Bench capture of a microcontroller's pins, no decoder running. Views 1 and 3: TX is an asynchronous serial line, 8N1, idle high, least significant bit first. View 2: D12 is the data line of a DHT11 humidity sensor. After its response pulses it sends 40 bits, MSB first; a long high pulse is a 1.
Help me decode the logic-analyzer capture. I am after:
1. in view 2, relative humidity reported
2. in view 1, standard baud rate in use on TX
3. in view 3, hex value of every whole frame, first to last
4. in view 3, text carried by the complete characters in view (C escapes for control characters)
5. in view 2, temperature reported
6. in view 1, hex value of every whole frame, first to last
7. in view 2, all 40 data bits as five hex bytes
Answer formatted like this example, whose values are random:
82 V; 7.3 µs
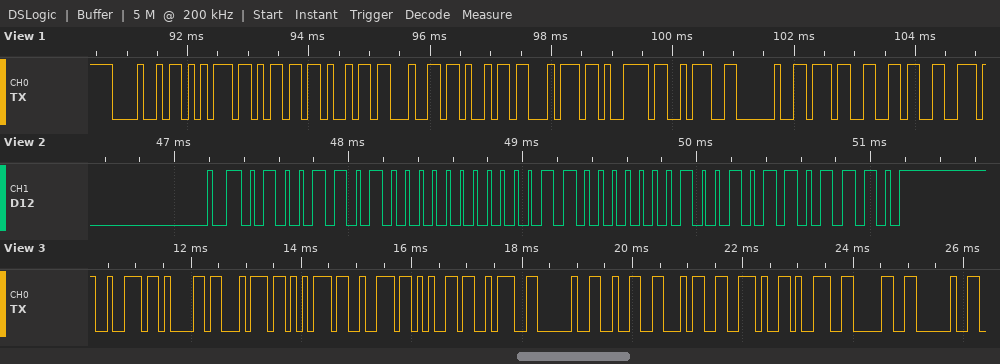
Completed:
77 %; 9600 baud; 0x72 0x61 0x74 0x75 0x72 0x65 0x3A 0x20 0x32 0x34 0x2E 0x39 0x30 0x20; "rature: 24.90 "; 24.9 °C; 0x48 0x75 0x6D 0x69 0x64 0x69 0x74 0x79 0x3A 0x20 0x37 0x36; 4D 00 18 09 6E
